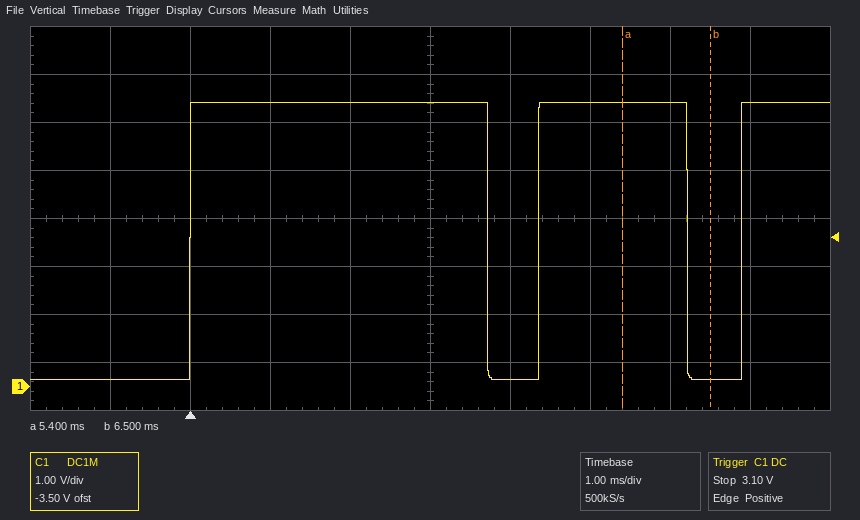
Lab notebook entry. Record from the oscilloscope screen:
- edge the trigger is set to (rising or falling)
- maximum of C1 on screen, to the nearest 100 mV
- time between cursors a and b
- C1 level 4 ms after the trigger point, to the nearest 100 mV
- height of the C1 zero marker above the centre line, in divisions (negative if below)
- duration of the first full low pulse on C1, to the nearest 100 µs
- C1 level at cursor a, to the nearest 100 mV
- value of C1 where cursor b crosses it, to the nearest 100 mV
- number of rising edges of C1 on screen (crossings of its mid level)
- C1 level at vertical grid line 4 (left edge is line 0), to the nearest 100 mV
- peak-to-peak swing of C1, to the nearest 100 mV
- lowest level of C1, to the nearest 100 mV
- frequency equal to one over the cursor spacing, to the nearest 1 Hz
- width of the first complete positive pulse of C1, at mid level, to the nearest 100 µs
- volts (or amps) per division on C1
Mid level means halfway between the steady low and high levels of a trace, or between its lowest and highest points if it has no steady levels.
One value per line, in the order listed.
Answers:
rising
5.9 V
1.1 ms
100 mV
-3.5 div
600 µs
5.9 V
100 mV
3
5.9 V
5.8 V
100 mV
909 Hz
3.7 ms
1 V
